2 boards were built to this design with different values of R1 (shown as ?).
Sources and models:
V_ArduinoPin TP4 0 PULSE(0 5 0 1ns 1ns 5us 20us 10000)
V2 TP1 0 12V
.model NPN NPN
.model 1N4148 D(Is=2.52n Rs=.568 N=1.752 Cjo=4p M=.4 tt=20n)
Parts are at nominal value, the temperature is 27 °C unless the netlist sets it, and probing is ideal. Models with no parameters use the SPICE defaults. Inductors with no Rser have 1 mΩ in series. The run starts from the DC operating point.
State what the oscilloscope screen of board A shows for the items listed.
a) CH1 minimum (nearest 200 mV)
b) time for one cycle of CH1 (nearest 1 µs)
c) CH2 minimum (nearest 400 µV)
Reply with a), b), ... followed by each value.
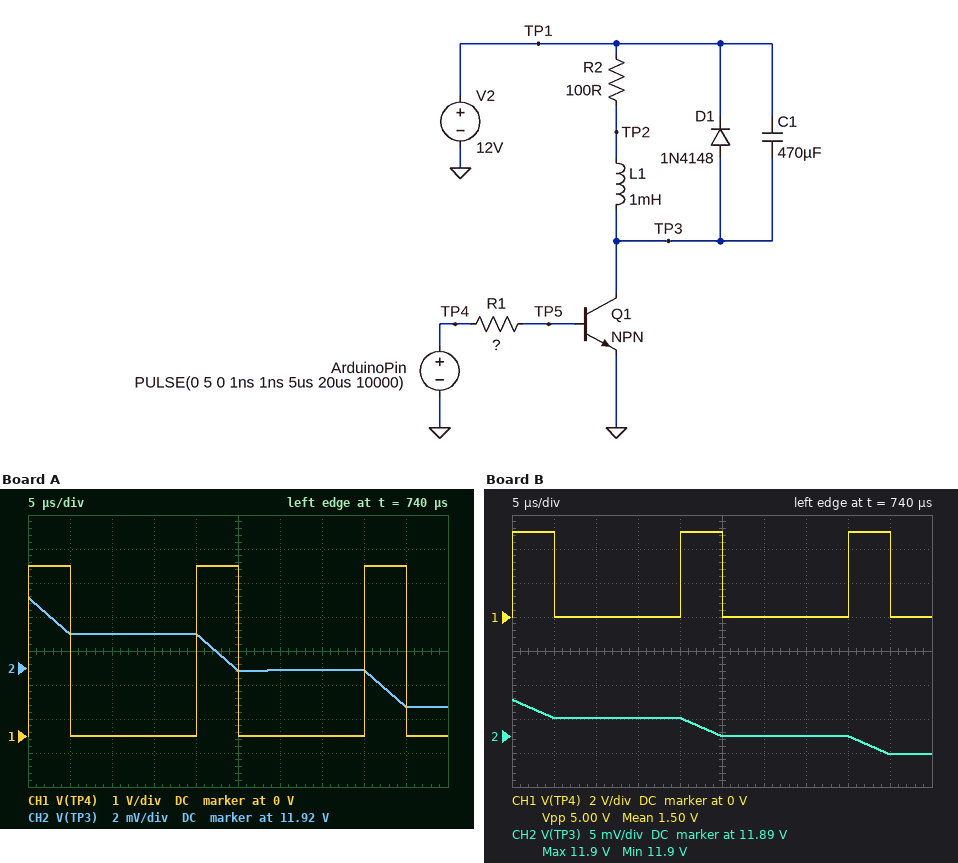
a) 0 V
b) 20 µs
c) 11.9136 V
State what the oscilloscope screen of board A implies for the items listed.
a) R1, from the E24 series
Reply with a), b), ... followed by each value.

a) 2 kΩ
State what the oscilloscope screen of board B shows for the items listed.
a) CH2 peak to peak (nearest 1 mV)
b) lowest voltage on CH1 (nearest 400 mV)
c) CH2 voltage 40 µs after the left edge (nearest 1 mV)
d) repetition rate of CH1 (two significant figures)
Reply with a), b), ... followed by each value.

a) 8 mV
b) 0 V
c) 11.895 V
d) 50 kHz
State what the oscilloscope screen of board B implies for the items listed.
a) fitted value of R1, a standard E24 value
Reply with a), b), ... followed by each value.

a) 1.6 kΩ
